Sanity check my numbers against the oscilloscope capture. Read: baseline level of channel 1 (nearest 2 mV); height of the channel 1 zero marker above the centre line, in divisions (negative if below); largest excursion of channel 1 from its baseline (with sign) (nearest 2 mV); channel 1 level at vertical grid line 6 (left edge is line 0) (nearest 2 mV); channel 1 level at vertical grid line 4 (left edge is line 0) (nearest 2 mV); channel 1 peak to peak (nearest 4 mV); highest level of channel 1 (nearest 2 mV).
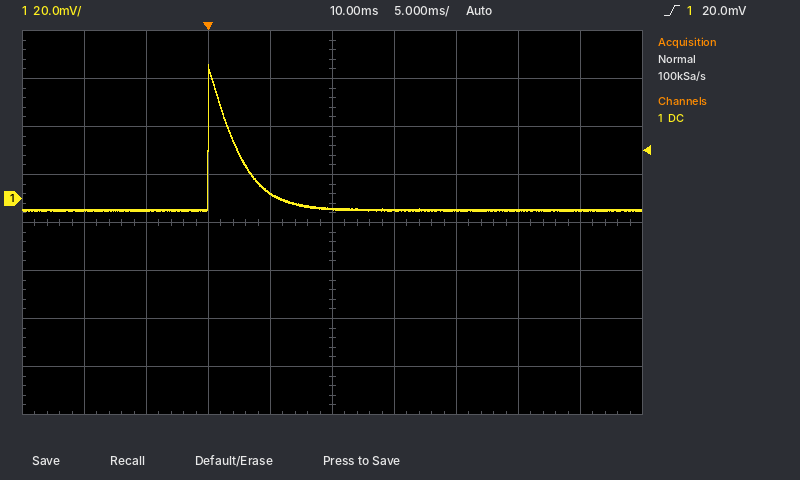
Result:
-4 mV
+0.5 div
+60 mV
-4 mV
2 mV
60 mV
56 mV
